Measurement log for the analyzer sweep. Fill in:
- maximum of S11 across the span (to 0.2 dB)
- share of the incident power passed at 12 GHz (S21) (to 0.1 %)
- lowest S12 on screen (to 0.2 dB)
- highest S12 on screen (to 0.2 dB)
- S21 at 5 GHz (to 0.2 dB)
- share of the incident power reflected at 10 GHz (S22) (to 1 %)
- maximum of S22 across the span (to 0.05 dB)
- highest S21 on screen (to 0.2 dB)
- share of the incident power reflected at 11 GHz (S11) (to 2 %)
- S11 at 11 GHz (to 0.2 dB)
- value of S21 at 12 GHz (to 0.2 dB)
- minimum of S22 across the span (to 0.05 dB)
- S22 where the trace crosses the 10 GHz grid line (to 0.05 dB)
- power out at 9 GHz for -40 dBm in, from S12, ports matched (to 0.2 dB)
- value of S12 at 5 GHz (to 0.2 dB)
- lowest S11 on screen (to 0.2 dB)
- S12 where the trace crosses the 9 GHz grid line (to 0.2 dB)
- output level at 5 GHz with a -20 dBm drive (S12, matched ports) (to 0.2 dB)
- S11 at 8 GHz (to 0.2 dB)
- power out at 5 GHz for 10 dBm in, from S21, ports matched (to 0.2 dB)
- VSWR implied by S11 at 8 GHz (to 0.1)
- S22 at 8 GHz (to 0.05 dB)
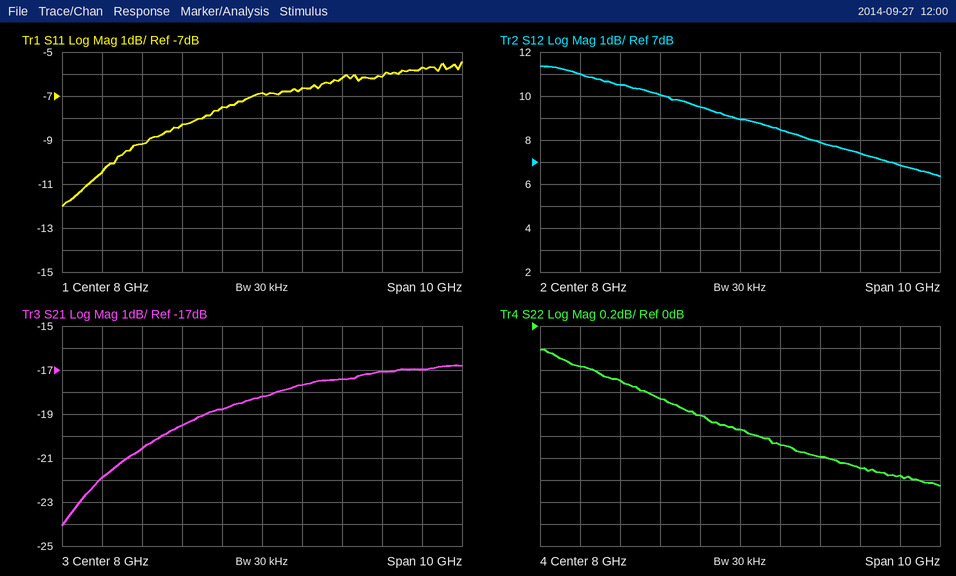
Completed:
-5.4 dB
2.0 %
6.4 dB
11.4 dB
-20.6 dB
76 %
-0.20 dB
-16.8 dB
24 %
-6.2 dB
-17.0 dB
-1.45 dB
-1.20 dB
-31.6 dBm
10.6 dB
-12.0 dB
8.4 dB
-9.4 dBm
-6.8 dB
-10.6 dBm
2.7
-0.95 dB
